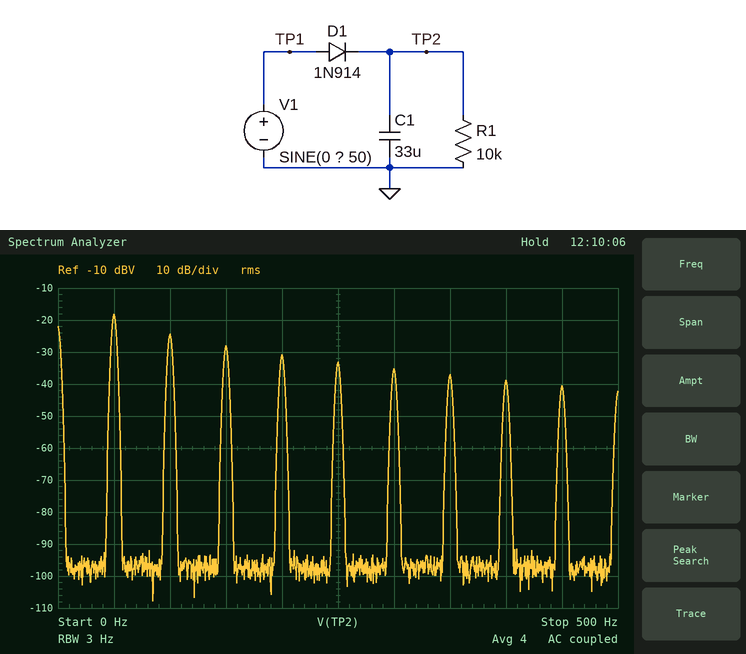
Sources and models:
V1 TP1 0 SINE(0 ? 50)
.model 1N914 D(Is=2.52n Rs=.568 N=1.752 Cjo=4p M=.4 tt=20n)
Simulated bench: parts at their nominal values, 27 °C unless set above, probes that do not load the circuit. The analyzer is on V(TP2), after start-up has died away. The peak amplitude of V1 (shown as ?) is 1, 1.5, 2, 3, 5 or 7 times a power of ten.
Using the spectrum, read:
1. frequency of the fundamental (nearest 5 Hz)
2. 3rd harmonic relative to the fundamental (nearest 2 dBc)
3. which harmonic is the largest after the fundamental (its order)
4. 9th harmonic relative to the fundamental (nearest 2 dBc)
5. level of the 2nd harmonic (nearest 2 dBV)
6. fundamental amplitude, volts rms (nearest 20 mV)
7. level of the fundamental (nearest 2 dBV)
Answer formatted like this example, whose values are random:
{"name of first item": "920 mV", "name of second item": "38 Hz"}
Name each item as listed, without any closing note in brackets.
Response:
{"frequency of the fundamental": "50 Hz", "3rd harmonic relative to the fundamental": "-10 dBc", "which harmonic is the largest after the fundamental": "2", "9th harmonic relative to the fundamental": "-22 dBc", "level of the 2nd harmonic": "-24 dBV", "fundamental amplitude, volts rms": "120 mV", "level of the fundamental": "-18 dBV"}
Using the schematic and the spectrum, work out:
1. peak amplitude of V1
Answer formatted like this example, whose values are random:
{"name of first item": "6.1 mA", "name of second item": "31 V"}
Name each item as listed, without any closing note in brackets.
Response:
{"peak amplitude of V1": "10 V"}
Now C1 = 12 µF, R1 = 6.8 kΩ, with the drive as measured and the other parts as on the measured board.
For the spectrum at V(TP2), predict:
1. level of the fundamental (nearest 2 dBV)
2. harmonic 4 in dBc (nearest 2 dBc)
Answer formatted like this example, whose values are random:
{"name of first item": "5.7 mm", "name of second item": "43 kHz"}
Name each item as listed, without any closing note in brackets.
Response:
{"level of the fundamental": "-6 dBV", "harmonic 4 in dBc": "-14 dBc"}
